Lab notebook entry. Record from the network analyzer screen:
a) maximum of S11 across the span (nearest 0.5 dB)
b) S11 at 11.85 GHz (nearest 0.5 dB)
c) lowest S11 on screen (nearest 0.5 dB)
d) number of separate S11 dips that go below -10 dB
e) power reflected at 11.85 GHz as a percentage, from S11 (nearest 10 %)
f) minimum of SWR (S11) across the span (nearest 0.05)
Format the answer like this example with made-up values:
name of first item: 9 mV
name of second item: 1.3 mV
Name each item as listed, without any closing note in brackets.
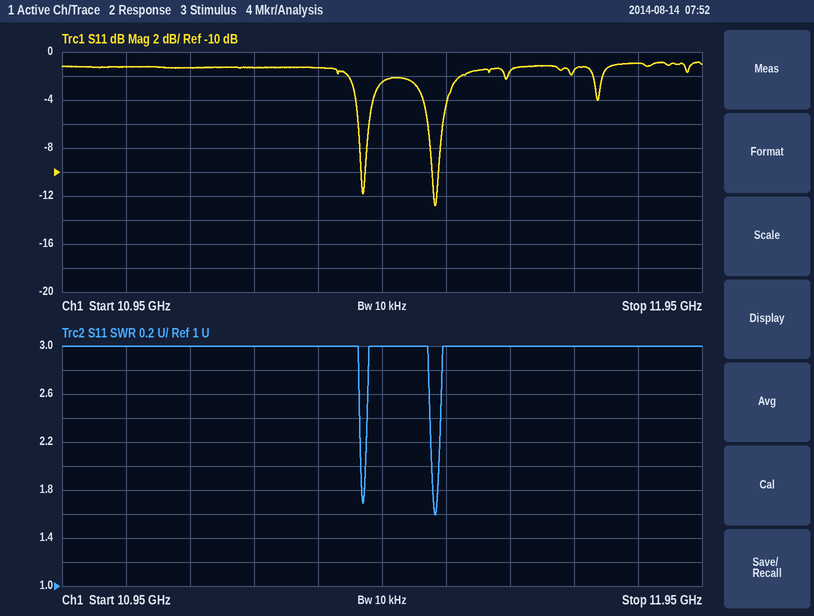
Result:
maximum of S11 across the span: -1.0 dB
S11 at 11.85 GHz: -1.0 dB
lowest S11 on screen: -13.0 dB
number of separate S11 dips that go below -10 dB: 2
power reflected at 11.85 GHz as a percentage, from S11: 80 %
minimum of SWR (S11) across the span: 1.60
